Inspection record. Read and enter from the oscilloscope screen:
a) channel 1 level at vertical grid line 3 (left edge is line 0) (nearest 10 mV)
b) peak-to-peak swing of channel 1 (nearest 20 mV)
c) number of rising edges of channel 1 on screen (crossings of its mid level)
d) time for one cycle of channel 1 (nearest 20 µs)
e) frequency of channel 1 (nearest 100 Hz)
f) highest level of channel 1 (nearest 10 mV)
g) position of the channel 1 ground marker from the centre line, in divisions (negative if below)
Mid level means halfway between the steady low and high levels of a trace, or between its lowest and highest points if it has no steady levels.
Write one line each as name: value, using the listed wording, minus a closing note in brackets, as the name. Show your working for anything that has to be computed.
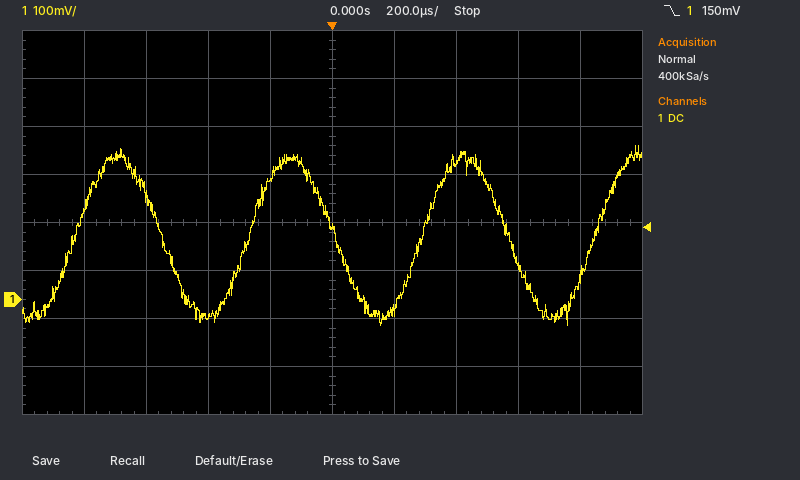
channel 1 level at vertical grid line 3 (left edge is line 0): -40 mV
peak-to-peak swing of channel 1: 380 mV
number of rising edges of channel 1 on screen: 4
time for one cycle of channel 1: 560 µs
frequency of channel 1: 1 / 560 µs ≈ 1.8 kHz
highest level of channel 1: 320 mV
position of the channel 1 ground marker from the centre line, in divisions: -1.6 div
